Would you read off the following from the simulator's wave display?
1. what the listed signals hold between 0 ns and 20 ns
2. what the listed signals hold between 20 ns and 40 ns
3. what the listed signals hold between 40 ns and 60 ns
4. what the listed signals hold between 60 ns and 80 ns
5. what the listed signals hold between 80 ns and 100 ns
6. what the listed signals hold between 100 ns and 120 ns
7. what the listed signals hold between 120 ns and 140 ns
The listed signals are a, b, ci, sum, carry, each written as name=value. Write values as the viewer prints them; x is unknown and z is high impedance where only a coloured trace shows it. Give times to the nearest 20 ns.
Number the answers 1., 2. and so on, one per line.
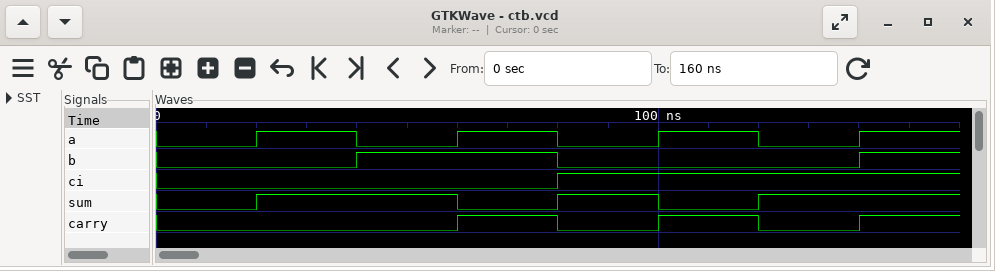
1. a=0, b=0, ci=0, sum=0, carry=0
2. a=1, b=0, ci=0, sum=1, carry=0
3. a=0, b=1, ci=0, sum=1, carry=0
4. a=1, b=1, ci=0, sum=0, carry=1
5. a=0, b=0, ci=1, sum=1, carry=0
6. a=1, b=0, ci=1, sum=0, carry=1
7. a=0, b=0, ci=1, sum=1, carry=0
